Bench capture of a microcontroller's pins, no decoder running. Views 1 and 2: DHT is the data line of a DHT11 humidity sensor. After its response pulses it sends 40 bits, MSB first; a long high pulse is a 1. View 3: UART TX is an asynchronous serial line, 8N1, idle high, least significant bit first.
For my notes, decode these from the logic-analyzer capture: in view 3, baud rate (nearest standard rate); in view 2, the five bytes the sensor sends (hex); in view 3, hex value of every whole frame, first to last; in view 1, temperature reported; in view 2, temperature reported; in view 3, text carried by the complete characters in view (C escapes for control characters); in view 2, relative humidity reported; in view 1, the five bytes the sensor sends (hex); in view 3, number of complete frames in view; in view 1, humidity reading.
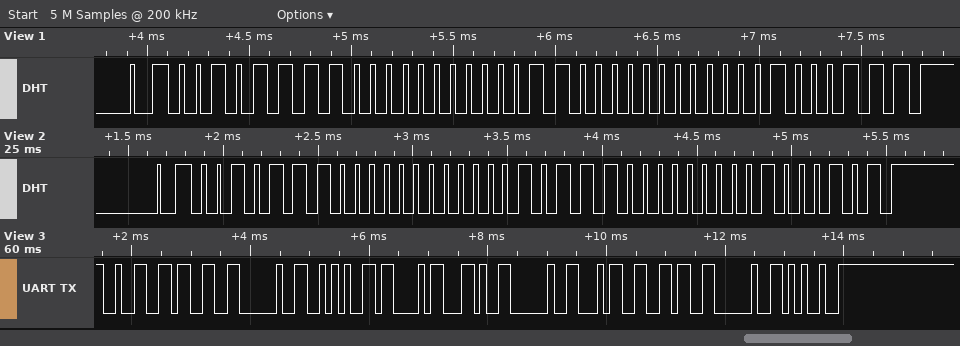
9600 baud
2E 00 17 00 45
32 33 20 2A 43 2C 20 34 36 20 25
24.0 °C
23.0 °C
"23 *C, 46 %"
46 %
2F 00 18 00 47
11
47 %
